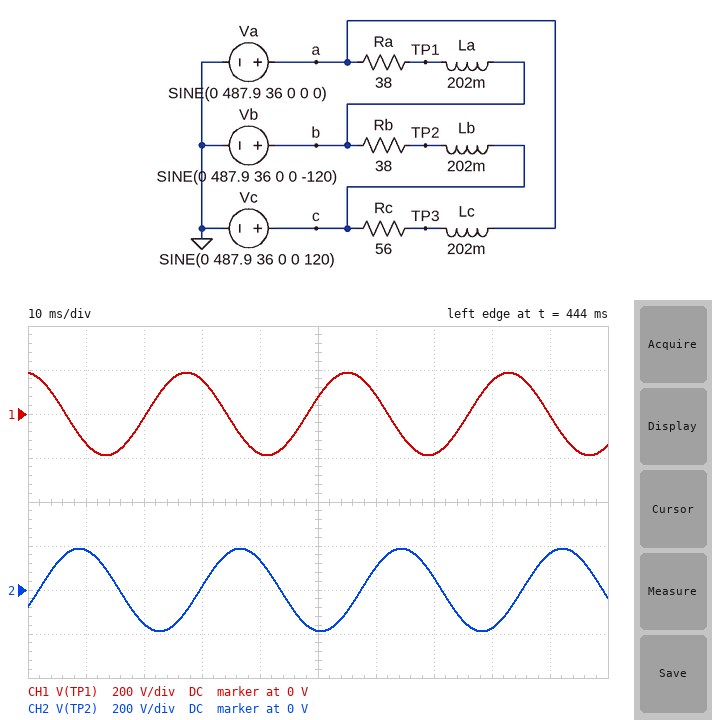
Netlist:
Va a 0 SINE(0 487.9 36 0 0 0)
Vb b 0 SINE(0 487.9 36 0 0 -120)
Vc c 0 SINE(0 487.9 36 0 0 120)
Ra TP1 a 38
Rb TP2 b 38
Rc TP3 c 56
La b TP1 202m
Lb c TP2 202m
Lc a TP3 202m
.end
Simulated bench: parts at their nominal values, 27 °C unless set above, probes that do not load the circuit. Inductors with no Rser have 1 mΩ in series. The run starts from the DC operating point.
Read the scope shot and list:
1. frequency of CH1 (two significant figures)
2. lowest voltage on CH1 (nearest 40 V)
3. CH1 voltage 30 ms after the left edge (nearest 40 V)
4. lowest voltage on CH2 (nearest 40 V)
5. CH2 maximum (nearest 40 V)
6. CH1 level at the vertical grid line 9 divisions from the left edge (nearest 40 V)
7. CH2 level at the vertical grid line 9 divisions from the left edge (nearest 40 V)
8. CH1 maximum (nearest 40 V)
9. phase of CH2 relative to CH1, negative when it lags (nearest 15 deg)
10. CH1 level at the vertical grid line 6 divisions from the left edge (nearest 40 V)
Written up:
36 Hz
-200 V
160 V
-200 V
200 V
0 V
160 V
200 V
-120 deg
80 V
